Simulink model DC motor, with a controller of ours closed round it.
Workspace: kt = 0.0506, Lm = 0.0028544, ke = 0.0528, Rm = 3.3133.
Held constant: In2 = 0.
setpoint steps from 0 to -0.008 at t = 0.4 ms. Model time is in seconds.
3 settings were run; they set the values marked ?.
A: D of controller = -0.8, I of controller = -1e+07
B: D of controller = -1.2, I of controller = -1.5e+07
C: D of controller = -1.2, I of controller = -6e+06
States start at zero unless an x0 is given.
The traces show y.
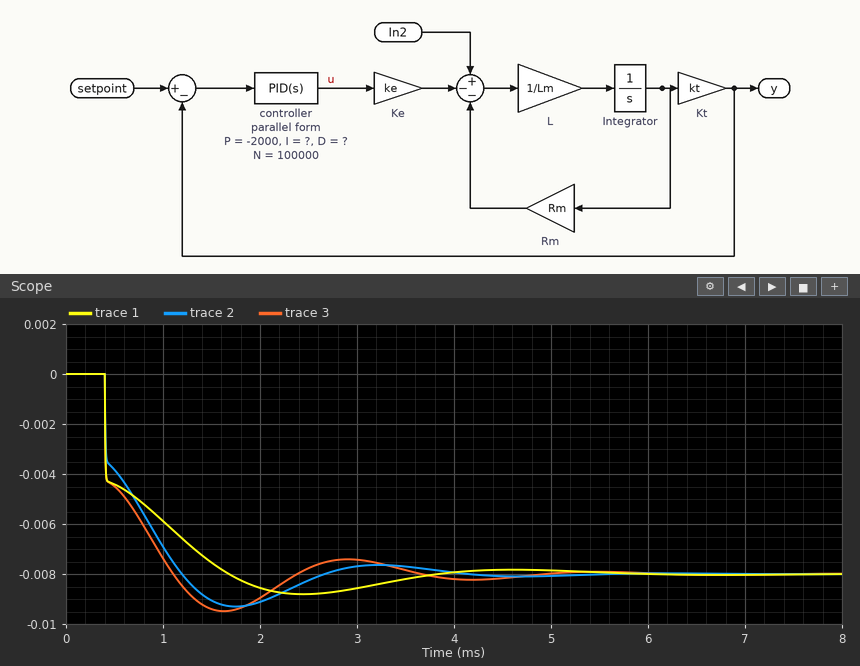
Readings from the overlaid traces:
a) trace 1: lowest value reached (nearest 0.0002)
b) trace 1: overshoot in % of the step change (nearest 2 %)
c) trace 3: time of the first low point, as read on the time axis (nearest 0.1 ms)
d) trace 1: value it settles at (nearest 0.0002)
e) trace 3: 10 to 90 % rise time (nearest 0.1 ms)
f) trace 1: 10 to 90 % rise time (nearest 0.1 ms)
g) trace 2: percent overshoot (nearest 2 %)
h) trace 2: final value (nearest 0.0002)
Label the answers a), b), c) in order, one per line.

a) -0.0088
b) 10 %
c) 1.6 ms
d) -0.0080
e) 0.6 ms
f) 1.0 ms
g) 16 %
h) -0.0080
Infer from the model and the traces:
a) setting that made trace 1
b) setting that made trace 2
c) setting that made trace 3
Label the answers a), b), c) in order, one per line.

a) C
b) A
c) B
